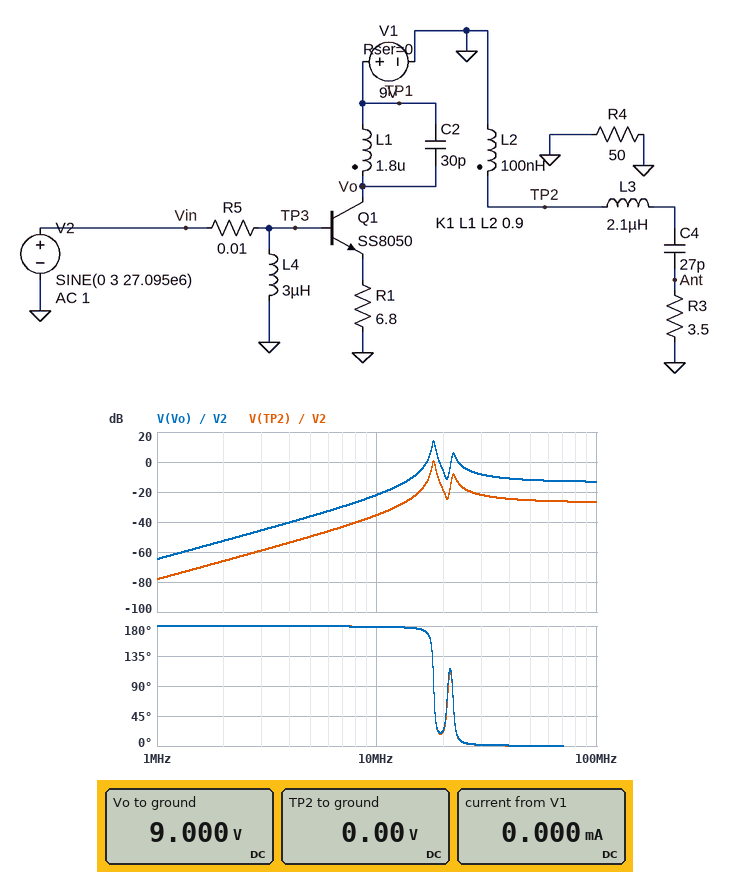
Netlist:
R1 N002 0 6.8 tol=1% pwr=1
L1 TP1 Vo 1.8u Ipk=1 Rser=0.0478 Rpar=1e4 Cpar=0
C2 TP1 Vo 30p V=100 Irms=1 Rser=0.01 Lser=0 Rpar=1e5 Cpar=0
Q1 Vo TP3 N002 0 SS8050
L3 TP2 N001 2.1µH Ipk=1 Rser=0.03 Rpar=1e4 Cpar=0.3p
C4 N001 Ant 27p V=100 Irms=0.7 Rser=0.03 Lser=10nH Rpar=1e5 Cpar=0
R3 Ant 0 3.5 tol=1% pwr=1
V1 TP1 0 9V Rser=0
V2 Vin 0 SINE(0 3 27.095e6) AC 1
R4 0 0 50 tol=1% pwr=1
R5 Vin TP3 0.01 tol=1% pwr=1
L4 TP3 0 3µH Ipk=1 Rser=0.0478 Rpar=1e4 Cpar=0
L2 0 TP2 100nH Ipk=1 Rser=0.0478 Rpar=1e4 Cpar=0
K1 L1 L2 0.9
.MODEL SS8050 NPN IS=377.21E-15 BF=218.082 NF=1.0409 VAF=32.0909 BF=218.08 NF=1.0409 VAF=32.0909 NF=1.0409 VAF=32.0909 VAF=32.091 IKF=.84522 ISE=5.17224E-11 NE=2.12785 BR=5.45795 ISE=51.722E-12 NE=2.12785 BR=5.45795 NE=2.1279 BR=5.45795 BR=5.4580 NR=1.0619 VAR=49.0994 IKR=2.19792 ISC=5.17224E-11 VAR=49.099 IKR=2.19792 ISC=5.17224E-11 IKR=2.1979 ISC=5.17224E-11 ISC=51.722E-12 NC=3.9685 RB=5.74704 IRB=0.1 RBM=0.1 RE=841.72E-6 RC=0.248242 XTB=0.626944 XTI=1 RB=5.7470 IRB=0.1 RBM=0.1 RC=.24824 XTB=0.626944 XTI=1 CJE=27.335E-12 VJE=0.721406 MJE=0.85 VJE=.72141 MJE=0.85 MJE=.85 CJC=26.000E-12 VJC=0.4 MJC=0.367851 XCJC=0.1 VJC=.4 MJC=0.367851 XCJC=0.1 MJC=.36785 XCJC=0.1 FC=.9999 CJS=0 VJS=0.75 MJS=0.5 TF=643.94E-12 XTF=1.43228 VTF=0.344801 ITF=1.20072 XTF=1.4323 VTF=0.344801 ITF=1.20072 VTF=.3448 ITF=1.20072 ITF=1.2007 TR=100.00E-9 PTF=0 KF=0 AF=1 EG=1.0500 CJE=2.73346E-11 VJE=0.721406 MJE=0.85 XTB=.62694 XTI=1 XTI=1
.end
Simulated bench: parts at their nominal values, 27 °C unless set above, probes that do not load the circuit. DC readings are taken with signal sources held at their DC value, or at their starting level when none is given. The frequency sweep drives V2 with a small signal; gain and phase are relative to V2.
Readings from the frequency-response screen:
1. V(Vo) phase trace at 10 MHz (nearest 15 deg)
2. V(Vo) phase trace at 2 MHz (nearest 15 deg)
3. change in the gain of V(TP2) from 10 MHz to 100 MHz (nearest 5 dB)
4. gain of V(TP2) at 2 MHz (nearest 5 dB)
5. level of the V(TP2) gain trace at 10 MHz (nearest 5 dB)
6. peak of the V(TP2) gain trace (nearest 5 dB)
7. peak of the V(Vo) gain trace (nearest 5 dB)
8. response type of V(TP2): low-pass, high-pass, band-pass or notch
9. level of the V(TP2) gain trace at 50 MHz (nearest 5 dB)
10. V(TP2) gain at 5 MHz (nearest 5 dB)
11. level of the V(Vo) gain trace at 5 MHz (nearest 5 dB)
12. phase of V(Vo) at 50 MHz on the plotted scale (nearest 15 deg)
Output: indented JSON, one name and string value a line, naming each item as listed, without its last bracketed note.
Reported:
{
  "V(Vo) phase trace at 10 MHz": "180 deg",
  "V(Vo) phase trace at 2 MHz": "180 deg",
  "change in the gain of V(TP2) from 10 MHz to 100 MHz": "10 dB",
  "gain of V(TP2) at 2 MHz": "-65 dB",
  "level of the V(TP2) gain trace at 10 MHz": "-35 dB",
  "peak of the V(TP2) gain trace": "0 dB",
  "peak of the V(Vo) gain trace": "15 dB",
  "response type of V(TP2): low-pass, high-pass, band-pass or notch": "high-pass",
  "level of the V(TP2) gain trace at 50 MHz": "-25 dB",
  "V(TP2) gain at 5 MHz": "-50 dB",
  "level of the V(Vo) gain trace at 5 MHz": "-35 dB",
  "phase of V(Vo) at 50 MHz on the plotted scale": "0 deg"
}
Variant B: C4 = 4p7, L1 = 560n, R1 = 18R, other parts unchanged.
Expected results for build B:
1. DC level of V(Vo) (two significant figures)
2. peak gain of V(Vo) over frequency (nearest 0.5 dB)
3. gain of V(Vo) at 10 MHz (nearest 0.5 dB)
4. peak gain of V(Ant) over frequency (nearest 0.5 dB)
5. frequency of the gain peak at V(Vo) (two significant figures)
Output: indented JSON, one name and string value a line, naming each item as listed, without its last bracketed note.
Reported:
{
  "DC level of V(Vo)": "9.0 V",
  "peak gain of V(Vo) over frequency": "21.5 dB",
  "gain of V(Vo) at 10 MHz": "-34.0 dB",
  "peak gain of V(Ant) over frequency": "-30.5 dB",
  "frequency of the gain peak at V(Vo)": "34 MHz"
}
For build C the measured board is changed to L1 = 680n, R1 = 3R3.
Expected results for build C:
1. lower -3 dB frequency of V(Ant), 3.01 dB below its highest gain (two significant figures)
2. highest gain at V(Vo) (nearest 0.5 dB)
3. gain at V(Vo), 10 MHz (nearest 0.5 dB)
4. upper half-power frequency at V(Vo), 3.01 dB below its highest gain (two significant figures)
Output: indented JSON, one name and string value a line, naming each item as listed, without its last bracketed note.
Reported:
{
  "lower -3 dB frequency of V(Ant), 3.01 dB below its highest gain": "32 MHz",
  "highest gain at V(Vo)": "20.0 dB",
  "gain at V(Vo), 10 MHz": "-32.0 dB",
  "upper half-power frequency at V(Vo), 3.01 dB below its highest gain": "33 MHz"
}
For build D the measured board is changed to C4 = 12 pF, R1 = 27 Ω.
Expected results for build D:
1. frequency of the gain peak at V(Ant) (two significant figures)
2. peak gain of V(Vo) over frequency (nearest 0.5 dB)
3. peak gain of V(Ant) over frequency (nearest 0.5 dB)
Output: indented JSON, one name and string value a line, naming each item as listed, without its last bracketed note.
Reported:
{
  "frequency of the gain peak at V(Ant)": "19 MHz",
  "peak gain of V(Vo) over frequency": "18.0 dB",
  "peak gain of V(Ant) over frequency": "-37.5 dB"
}
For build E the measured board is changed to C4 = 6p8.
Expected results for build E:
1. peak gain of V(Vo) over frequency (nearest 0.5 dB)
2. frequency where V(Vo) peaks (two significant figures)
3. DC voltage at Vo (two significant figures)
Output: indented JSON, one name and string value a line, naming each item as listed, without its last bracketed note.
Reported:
{
  "peak gain of V(Vo) over frequency": "18.5 dB",
  "frequency where V(Vo) peaks": "19 MHz",
  "DC voltage at Vo": "9.0 V"
}
